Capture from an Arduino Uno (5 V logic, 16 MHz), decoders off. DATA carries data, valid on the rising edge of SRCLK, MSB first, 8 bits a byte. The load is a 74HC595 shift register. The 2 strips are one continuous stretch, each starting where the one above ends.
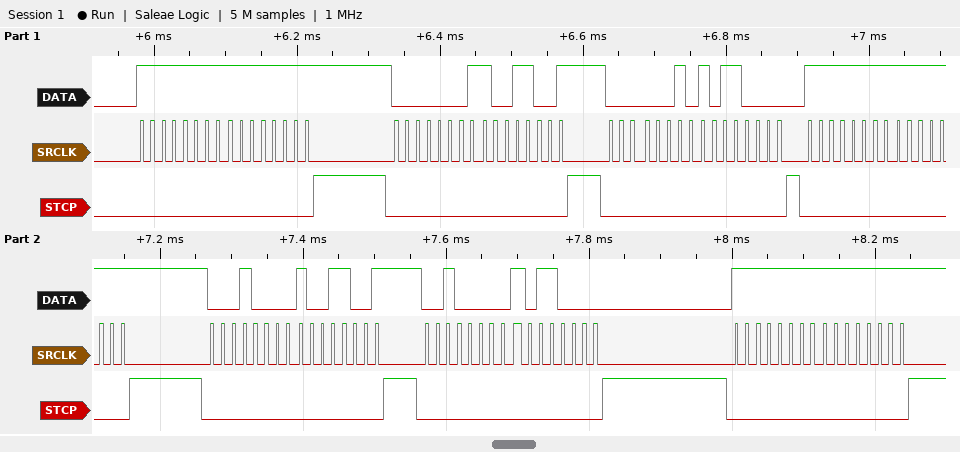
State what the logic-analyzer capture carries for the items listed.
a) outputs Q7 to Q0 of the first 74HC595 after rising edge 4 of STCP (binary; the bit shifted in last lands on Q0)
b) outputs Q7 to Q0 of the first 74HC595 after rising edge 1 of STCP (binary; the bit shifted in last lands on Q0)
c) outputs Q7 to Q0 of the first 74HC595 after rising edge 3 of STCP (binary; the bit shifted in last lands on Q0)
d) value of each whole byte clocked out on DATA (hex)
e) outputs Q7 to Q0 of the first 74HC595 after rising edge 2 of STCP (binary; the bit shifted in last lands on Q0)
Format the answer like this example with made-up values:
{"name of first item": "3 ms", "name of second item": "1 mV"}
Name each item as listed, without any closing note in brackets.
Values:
{"outputs Q7 to Q0 of the first 74HC595 after rising edge 4 of STCP": "11111111", "outputs Q7 to Q0 of the first 74HC595 after rising edge 1 of STCP": "11111111", "outputs Q7 to Q0 of the first 74HC595 after rising edge 3 of STCP": "10110000", "value of each whole byte clocked out on DATA": "FF FF 01 99 02 B0 FF FF 10 99 20 B0 FF FF", "outputs Q7 to Q0 of the first 74HC595 after rising edge 2 of STCP": "10011001"}
